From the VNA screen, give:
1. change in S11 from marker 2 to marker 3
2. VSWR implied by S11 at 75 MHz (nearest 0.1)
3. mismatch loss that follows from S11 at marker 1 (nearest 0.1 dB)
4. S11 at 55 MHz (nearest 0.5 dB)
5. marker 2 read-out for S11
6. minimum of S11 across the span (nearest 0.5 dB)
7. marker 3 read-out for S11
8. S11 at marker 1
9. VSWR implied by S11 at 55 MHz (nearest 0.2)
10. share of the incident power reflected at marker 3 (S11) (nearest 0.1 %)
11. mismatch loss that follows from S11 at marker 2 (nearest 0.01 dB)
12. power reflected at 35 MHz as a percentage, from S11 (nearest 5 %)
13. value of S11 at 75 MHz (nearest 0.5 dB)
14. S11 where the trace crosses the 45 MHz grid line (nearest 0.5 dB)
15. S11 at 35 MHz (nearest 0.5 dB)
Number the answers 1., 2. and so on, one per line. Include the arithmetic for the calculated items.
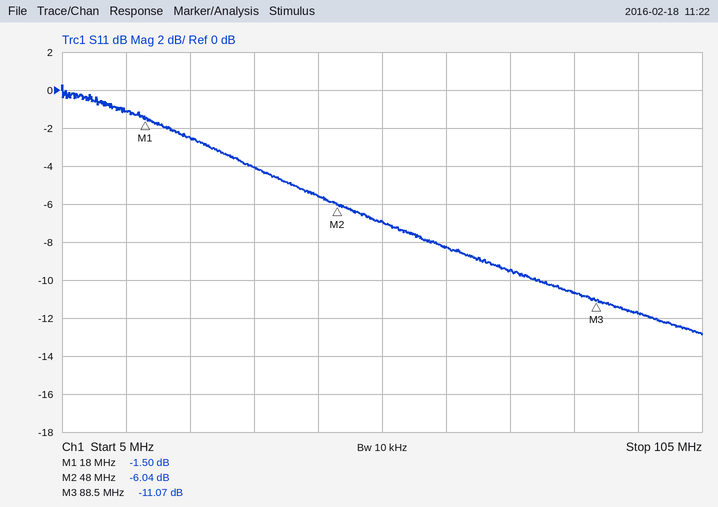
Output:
1. -11.07 − (-6.04) = -5.03 dB
2. |Γ| = 10^(-9.5/20) = 0.3350; VSWR = (1 + 0.3350)/(1 − 0.3350) ≈ 2.0
3. −10 log10(1 − 10^(-1.5/10)) ≈ 5.3 dB
4. -7.0 dB
5. -6.04 dB
6. -13.0 dB
7. -11.07 dB
8. -1.50 dB
9. |Γ| = 10^(-7/20) = 0.4467; VSWR = (1 + 0.4467)/(1 − 0.4467) ≈ 2.6
10. 10^(-11.07/10) ≈ 7.8 %
11. −10 log10(1 − 10^(-6.04/10)) ≈ 1.24 dB
12. 10^(-4/10) ≈ 40 %
13. -9.5 dB
14. -5.5 dB
15. -4.0 dB
